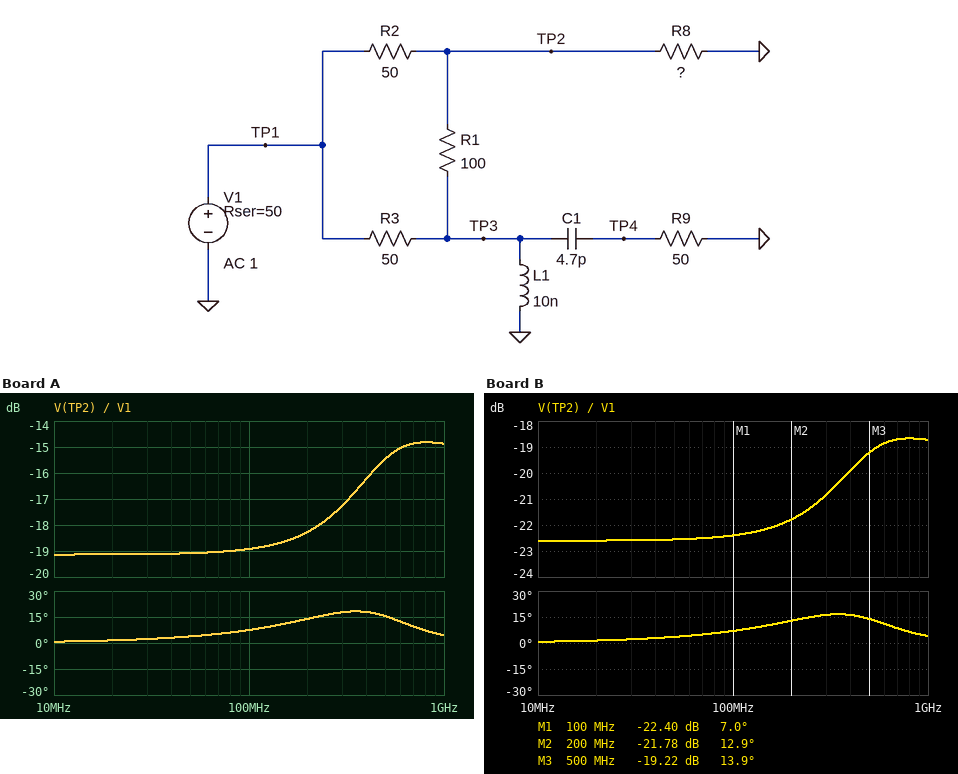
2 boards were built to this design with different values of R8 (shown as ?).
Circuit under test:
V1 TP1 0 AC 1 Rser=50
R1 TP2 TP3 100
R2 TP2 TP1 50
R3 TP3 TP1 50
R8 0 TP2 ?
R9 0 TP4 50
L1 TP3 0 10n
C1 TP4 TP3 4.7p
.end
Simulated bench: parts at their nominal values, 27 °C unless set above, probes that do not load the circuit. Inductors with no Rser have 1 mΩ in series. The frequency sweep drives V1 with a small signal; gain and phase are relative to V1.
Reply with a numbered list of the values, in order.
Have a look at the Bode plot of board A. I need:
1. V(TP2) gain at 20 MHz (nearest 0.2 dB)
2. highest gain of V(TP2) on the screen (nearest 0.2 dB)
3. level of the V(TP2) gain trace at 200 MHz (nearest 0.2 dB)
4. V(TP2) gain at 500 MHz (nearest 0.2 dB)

1. -19.2 dB
2. -14.8 dB
3. -18.2 dB
4. -15.4 dB
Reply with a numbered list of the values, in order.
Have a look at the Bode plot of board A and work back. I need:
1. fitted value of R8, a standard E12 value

1. 27 Ω
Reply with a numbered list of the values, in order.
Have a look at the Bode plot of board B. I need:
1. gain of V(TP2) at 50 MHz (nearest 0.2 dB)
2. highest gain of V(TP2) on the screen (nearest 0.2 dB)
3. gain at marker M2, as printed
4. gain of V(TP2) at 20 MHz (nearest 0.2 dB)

1. -22.6 dB
2. -18.6 dB
3. -21.78 dB
4. -22.6 dB
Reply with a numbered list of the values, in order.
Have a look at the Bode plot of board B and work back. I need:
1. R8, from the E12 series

1. 15 Ω
